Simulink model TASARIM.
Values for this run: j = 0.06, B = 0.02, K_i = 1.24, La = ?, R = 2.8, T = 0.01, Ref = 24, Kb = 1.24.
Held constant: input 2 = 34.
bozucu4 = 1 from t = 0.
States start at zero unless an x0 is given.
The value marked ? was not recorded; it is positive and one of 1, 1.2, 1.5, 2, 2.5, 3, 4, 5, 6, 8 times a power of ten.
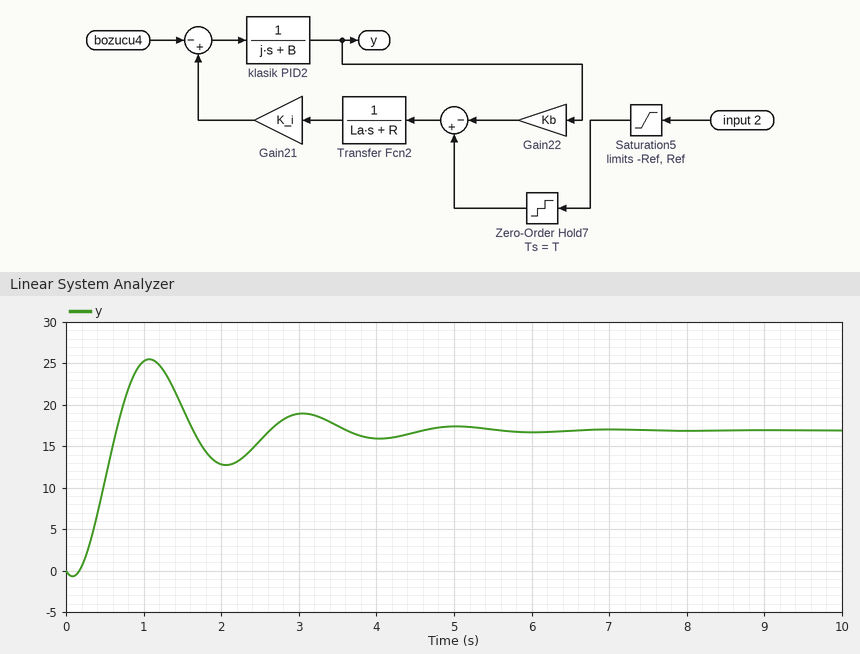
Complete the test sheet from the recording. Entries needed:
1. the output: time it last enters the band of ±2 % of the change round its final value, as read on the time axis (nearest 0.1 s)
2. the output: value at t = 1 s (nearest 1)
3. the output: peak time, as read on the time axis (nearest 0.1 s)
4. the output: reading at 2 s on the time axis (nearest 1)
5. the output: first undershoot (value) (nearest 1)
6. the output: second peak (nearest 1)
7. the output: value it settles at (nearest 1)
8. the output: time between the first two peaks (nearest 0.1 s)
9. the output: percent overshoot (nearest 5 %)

5.3 s
25
1.1 s
13
13
19
17
2.0 s
50 %
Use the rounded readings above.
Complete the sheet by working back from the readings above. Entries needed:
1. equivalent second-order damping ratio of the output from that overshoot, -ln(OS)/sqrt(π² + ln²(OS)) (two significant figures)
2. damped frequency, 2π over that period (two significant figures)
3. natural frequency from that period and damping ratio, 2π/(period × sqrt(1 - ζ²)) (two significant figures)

0.22
3.1 rad/s
3.2 rad/s
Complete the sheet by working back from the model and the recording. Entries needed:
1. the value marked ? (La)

2.5
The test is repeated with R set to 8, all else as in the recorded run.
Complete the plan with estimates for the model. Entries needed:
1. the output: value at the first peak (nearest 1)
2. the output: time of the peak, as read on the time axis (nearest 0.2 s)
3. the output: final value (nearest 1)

15
1.2 s
13
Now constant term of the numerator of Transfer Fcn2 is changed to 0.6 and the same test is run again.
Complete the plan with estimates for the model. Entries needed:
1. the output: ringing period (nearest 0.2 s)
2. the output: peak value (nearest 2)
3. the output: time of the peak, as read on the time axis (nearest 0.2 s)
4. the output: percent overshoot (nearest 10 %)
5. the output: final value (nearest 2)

2.6 s
22
1.4 s
40 %
16
